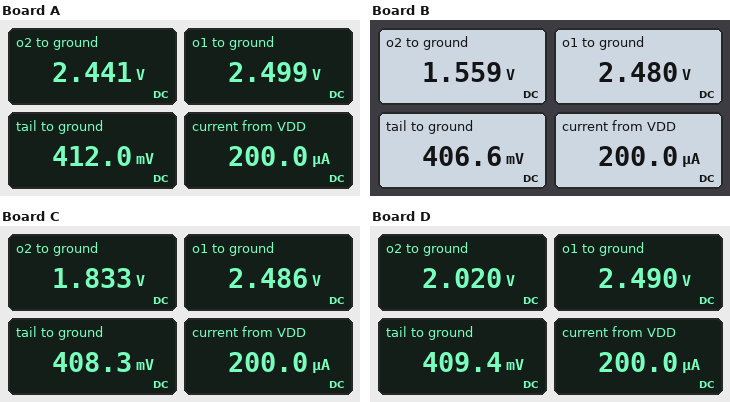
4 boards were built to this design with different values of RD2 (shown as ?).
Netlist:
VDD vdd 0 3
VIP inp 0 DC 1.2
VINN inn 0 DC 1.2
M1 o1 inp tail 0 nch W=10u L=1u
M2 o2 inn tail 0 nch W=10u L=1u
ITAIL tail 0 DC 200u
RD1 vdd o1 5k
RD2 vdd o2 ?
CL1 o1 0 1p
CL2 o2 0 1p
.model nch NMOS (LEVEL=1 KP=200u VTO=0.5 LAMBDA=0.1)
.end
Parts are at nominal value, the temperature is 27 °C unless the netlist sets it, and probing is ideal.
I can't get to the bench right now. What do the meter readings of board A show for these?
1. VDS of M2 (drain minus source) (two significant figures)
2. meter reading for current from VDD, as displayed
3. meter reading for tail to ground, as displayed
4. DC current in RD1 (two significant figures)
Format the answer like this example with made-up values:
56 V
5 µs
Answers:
2.0 V
200.0 µA
412.0 mV
100 µA
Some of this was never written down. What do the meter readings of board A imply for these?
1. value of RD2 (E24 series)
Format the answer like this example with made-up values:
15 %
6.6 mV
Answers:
5.6 kΩ
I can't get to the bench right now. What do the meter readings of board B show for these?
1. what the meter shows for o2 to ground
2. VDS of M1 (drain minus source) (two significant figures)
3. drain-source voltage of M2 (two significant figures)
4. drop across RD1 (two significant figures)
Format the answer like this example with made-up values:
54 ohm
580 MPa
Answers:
1.559 V
2.1 V
1.2 V
520 mV
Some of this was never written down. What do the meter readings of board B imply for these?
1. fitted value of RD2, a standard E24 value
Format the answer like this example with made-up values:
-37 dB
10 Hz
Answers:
15 kΩ
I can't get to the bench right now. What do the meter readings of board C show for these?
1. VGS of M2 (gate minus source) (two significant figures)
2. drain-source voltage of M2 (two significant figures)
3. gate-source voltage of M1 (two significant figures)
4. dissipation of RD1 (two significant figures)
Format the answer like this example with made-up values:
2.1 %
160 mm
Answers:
790 mV
1.4 V
790 mV
53 µW
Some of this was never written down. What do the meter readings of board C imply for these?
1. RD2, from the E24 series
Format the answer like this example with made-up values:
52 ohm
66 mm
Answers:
12 kΩ
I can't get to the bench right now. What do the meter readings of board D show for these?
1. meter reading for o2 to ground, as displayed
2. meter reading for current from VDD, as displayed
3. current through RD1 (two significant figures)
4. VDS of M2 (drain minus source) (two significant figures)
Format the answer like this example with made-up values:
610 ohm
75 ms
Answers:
2.020 V
200.0 µA
100 µA
1.6 V
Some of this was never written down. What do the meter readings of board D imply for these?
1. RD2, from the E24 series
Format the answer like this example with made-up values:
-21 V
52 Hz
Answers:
10 kΩ
